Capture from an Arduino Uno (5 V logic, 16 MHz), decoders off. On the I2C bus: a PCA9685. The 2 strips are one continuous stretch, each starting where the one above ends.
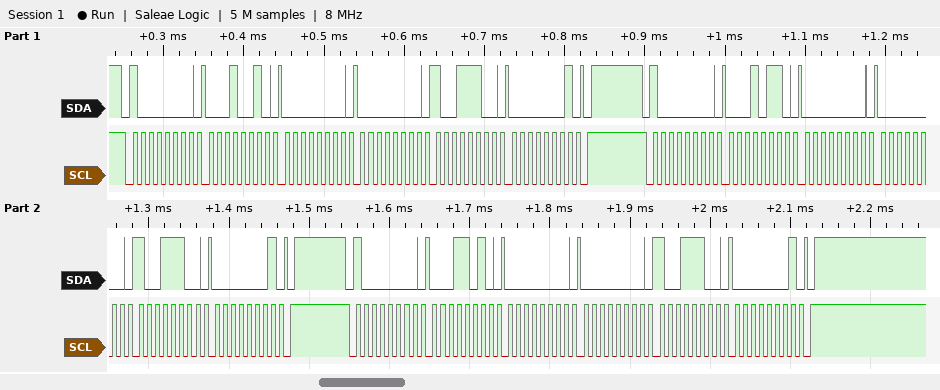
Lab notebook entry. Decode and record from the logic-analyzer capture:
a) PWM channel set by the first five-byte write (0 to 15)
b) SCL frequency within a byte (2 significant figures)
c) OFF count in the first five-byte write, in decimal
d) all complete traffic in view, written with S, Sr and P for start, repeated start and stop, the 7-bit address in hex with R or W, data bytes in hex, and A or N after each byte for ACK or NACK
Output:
3
100 kHz
412
S 40W A 12 A 00 A 00 A 9C A 01 A P S 40W A 16 A 00 A 00 A 9C A 01 A P S 40W A 1A A 00 A 00 A 9C A 01 A P
